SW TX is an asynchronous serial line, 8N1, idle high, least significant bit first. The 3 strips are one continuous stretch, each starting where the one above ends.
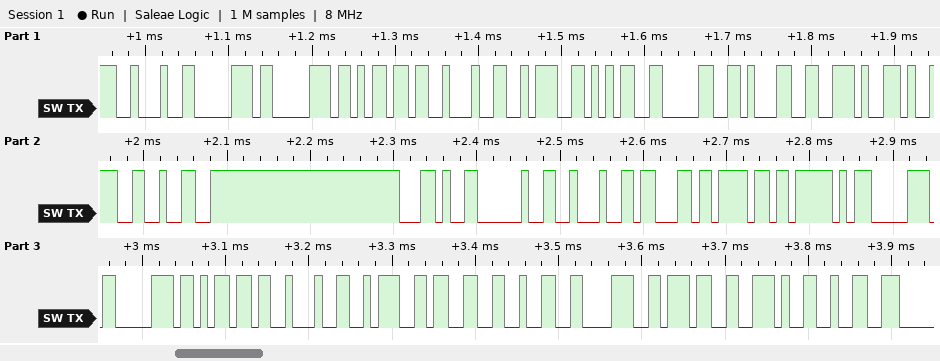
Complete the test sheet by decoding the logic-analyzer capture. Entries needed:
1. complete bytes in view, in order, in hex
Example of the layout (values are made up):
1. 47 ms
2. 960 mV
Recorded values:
1. 0x22 0x70 0x70 0x6D 0x22 0x3A 0x35 0x30 0x31 0x2E 0x39 0x32 0x2C 0x20 0x22 0x63 0x6F 0x5F 0x70 0x70 0x6D 0x22 0x3A 0x33 0x32 0x38 0x37 0x2E 0x32
